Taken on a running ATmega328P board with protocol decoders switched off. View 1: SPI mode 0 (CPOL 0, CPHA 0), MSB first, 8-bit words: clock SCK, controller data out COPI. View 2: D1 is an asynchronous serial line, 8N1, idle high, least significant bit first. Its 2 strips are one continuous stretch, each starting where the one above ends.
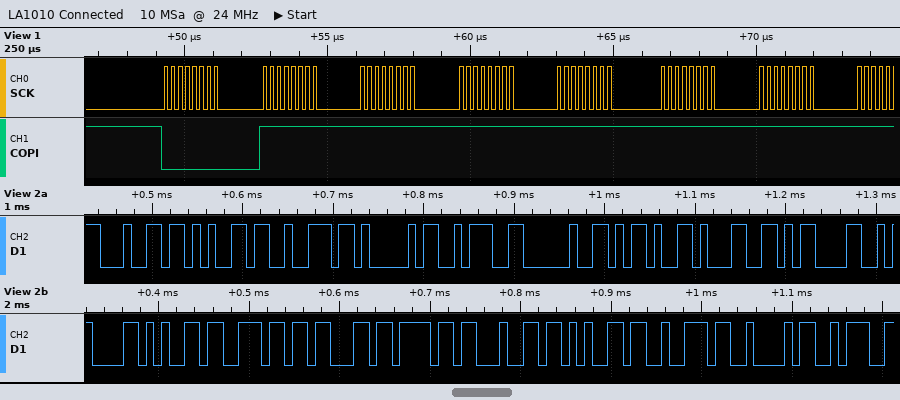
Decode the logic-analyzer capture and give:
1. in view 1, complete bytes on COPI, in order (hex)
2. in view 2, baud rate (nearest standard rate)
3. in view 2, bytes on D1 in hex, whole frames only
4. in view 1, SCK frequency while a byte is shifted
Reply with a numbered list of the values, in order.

1. 00 FF FF FF FF FF FF
2. 115200 baud
3. 0x64 0x65 0x72 0x41 0x3A 0x20 0x2D 0x31 0x0D 0x0A 0x65 0x6E 0x63 0x6F 0x64 0x65 0x72 0x42 0x3A
4. 4 MHz
